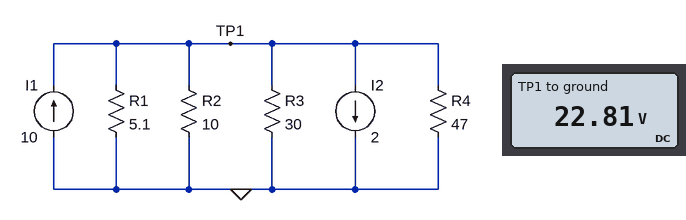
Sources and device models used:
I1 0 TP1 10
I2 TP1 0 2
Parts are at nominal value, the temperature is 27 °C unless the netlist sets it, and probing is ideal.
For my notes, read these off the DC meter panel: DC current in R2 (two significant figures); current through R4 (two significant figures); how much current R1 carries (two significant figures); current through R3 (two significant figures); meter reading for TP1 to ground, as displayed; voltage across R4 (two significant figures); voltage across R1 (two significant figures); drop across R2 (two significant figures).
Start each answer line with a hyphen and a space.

- 2.3 A
- 490 mA
- 4.5 A
- 760 mA
- 22.81 V
- 23 V
- 23 V
- 23 V
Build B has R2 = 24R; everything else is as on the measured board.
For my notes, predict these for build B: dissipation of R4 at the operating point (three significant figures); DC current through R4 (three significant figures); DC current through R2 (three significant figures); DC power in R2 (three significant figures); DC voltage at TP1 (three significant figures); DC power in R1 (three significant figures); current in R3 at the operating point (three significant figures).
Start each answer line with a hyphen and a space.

- 15.9 W
- 582 mA
- 1.14 A
- 31.2 W
- 27.4 V
- 147 W
- 912 mA
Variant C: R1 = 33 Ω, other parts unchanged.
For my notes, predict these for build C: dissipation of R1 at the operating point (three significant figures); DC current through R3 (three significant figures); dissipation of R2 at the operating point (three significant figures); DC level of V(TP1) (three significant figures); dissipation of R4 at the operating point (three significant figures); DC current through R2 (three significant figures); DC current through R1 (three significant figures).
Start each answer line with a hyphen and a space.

- 56.7 W
- 1.44 A
- 187 W
- 43.3 V
- 39.8 W
- 4.33 A
- 1.31 A
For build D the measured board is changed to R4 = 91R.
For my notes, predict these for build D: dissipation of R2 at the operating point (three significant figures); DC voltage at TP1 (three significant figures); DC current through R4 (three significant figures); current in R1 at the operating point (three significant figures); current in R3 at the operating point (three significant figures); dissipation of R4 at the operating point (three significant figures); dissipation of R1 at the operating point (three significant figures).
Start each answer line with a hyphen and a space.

- 55.2 W
- 23.5 V
- 258 mA
- 4.61 A
- 783 mA
- 6.07 W
- 108 W
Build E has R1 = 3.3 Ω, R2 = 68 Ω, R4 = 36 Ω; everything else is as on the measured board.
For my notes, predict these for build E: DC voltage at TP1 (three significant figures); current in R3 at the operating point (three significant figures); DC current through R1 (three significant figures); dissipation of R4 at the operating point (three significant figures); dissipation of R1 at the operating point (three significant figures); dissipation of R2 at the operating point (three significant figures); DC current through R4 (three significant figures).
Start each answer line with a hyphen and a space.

- 21.1 V
- 704 mA
- 6.40 A
- 12.4 W
- 135 W
- 6.56 W
- 587 mA
